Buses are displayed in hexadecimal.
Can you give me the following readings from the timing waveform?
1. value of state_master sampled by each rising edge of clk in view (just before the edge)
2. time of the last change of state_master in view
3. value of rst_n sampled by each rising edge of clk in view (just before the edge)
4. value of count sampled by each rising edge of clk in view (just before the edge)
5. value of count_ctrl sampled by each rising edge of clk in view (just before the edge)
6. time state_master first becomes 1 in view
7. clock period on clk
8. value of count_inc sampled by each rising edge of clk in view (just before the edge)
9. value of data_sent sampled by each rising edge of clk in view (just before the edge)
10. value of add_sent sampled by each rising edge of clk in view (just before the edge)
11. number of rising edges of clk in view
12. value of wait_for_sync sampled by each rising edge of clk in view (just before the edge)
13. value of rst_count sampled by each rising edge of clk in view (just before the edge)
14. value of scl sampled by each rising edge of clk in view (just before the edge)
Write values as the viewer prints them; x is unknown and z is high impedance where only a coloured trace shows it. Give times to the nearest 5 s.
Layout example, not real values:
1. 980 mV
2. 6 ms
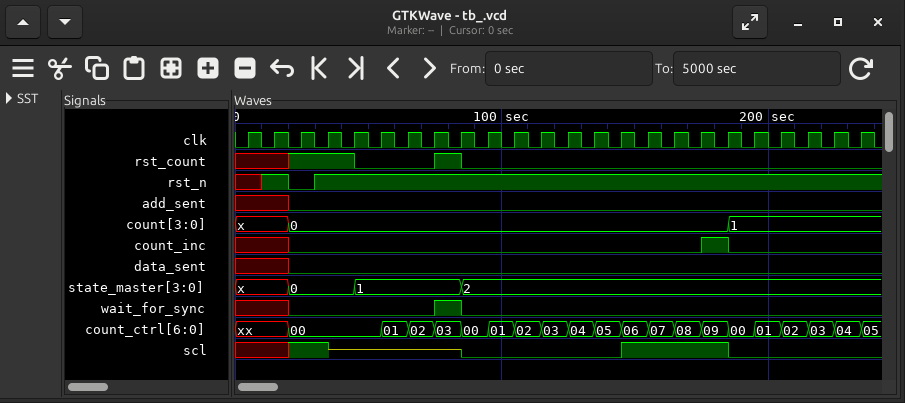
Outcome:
1. x, x, 0, 0, 0, 1, 1, 1, 1, 2, 2, 2, 2, 2, 2, 2, 2, 2, 2, 2, 2, 2, 2, 2
2. 85 s
3. x 1 0 1 1 1 1 1 1 1 1 1 1 1 1 1 1 1 1 1 1 1 1 1
4. x, x, 0, 0, 0, 0, 0, 0, 0, 0, 0, 0, 0, 0, 0, 0, 0, 0, 0, 1, 1, 1, 1, 1
5. xx, xx, 00, 00, 00, 00, 01, 02, 03, 00, 01, 02, 03, 04, 05, 06, 07, 08, 09, 00, 01, 02, 03, 04
6. 45 s
7. 10 s
8. x x 0 0 0 0 0 0 0 0 0 0 0 0 0 0 0 0 1 0 0 0 0 0
9. x x 0 0 0 0 0 0 0 0 0 0 0 0 0 0 0 0 0 0 0 0 0 0
10. x x 0 0 0 0 0 0 0 0 0 0 0 0 0 0 0 0 0 0 0 0 0 0
11. 24
12. x x 0 0 0 0 0 0 1 0 0 0 0 0 0 0 0 0 0 0 0 0 0 0
13. x x 1 1 1 0 0 0 1 0 0 0 0 0 0 0 0 0 0 0 0 0 0 0
14. x x 1 1 z z z z z 0 0 0 0 0 0 1 1 1 1 0 0 0 0 0
